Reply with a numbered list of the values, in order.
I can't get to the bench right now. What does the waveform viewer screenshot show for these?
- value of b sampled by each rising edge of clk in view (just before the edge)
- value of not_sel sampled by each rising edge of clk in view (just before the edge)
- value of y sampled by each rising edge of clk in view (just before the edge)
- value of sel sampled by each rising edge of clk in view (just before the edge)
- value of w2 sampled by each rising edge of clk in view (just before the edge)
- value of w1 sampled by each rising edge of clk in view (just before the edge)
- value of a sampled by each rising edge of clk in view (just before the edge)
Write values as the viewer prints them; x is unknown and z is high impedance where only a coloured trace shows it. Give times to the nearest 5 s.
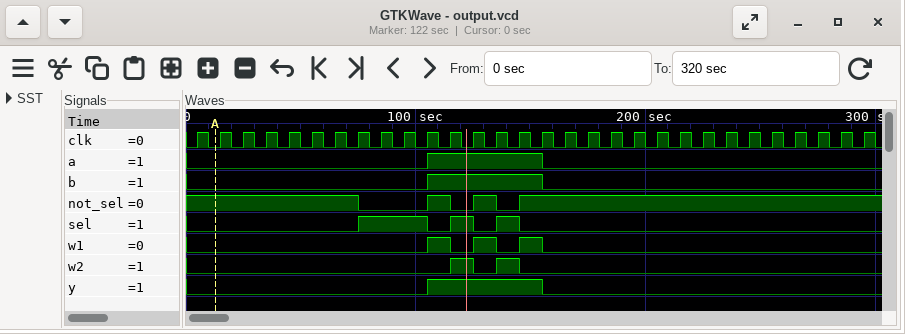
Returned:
1. 0 0 0 0 0 0 0 0 0 0 0 1 1 1 1 1 0 0 0 0 0 0 0 0 0 0 0 0 0 0
2. 1 1 1 1 1 1 1 1 0 0 0 1 0 1 0 1 1 1 1 1 1 1 1 1 1 1 1 1 1 1
3. 0 0 0 0 0 0 0 0 0 0 0 1 1 1 1 1 0 0 0 0 0 0 0 0 0 0 0 0 0 0
4. 0 0 0 0 0 0 0 0 1 1 1 0 1 0 1 0 0 0 0 0 0 0 0 0 0 0 0 0 0 0
5. 0 0 0 0 0 0 0 0 0 0 0 0 1 0 1 0 0 0 0 0 0 0 0 0 0 0 0 0 0 0
6. 0 0 0 0 0 0 0 0 0 0 0 1 0 1 0 1 0 0 0 0 0 0 0 0 0 0 0 0 0 0
7. 0 0 0 0 0 0 0 0 0 0 0 1 1 1 1 1 0 0 0 0 0 0 0 0 0 0 0 0 0 0
